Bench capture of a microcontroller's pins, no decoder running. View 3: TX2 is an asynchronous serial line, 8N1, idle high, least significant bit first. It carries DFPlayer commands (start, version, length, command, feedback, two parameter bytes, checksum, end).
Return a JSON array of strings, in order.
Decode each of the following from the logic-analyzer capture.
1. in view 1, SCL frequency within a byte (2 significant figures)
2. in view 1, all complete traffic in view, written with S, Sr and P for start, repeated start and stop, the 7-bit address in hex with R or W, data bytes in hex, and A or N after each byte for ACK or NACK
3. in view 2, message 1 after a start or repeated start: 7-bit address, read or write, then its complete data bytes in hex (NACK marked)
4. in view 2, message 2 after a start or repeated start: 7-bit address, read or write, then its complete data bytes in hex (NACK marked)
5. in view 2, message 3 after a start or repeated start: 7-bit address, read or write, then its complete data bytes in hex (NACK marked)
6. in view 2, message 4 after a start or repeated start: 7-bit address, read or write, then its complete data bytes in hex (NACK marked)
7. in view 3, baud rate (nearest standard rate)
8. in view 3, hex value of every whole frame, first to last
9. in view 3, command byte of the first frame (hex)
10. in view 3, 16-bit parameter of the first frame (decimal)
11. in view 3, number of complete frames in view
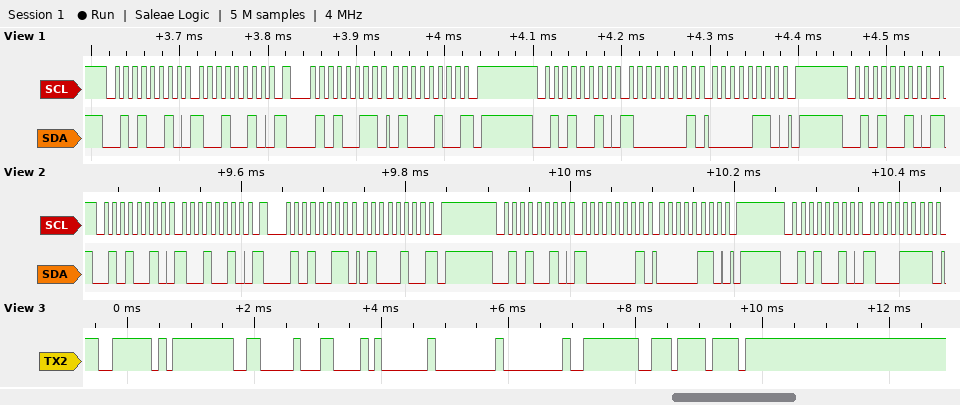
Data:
["100 kHz", "S 29W A 92 A Sr 29R A 44 N P S 29W A 81 A 06 A P S 29W A", "0x29 write: 92", "0x29 read: 44 NACK", "0x29 write: 81 06", "0x29 write: 8F", "9600 baud", "7E FF 06 0C 01 00 00 FE EE EF", "0x0C", "0", "10"]
